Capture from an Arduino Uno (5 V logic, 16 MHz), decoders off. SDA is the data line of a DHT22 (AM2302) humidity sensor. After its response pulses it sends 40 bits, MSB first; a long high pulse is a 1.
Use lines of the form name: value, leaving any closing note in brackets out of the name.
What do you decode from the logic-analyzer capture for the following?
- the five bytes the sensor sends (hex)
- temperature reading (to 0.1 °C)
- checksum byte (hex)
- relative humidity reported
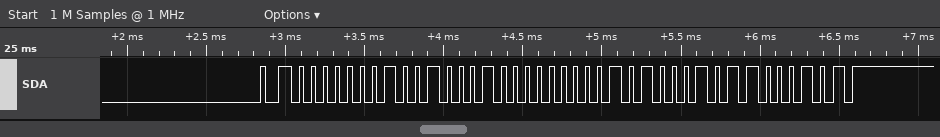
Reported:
the five bytes the sensor sends: 01 22 00 A2 C5
temperature reading: 16.2 °C
checksum byte: 0xC5
relative humidity reported: 29.0 %
